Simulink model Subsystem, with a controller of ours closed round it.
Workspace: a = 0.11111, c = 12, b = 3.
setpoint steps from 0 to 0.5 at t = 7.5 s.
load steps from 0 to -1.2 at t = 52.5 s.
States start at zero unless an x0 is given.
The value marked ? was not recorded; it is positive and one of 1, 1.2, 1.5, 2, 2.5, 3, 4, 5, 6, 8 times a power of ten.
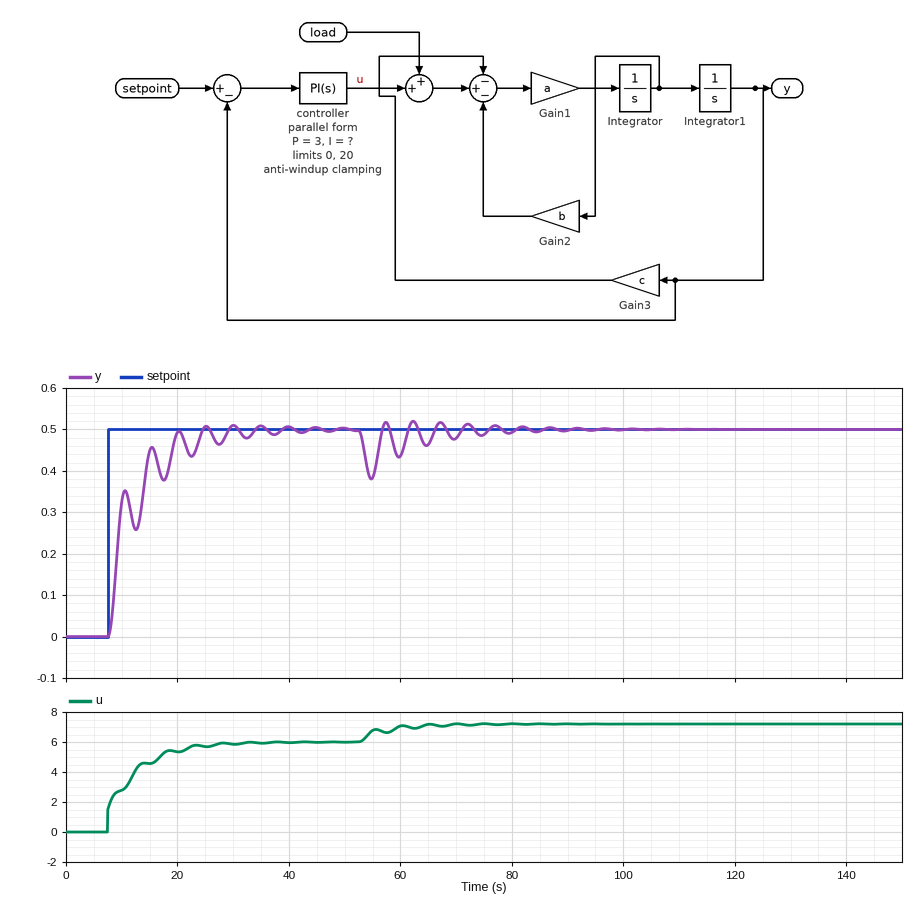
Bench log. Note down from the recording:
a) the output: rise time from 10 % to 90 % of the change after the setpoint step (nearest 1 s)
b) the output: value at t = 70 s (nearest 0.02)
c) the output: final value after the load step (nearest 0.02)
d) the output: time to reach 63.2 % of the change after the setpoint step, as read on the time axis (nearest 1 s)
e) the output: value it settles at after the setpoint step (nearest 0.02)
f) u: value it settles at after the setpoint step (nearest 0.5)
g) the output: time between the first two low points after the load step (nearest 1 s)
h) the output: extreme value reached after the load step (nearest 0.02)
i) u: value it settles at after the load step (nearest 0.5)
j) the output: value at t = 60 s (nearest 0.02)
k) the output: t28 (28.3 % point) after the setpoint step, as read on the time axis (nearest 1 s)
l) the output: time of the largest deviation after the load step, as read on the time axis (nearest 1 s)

7 s
0.48
0.50
10 s
0.50
6.0
5 s
0.38
7.0
0.44
9 s
55 s
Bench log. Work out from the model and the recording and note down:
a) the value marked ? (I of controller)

2.5
